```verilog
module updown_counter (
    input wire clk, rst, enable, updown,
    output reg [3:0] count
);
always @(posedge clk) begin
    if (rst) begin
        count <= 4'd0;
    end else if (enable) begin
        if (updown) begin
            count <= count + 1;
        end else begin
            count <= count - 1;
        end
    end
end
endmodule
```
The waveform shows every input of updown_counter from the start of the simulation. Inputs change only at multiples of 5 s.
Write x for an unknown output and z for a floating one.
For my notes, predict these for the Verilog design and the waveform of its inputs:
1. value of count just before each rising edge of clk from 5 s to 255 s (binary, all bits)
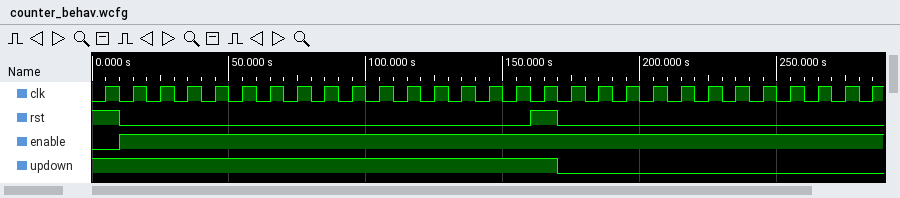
x, 0000, 0001, 0010, 0011, 0100, 0101, 0110, 0111, 1000, 1001, 1010, 1011, 1100, 1101, 1110, 1111, 0000, 1111, 1110, 1101, 1100, 1011, 1010, 1001, 1000
